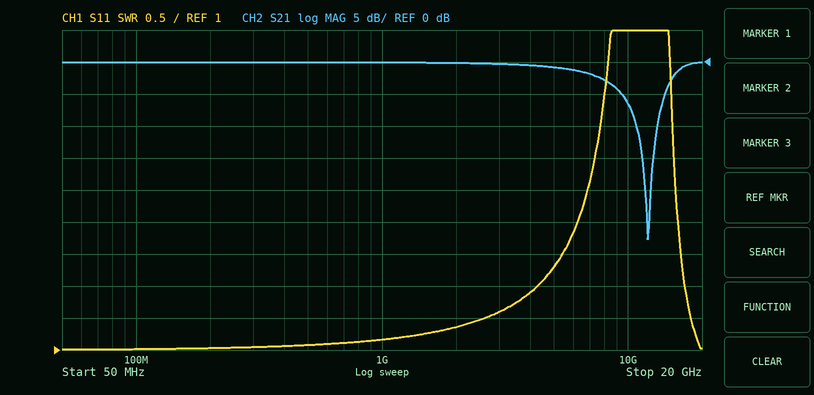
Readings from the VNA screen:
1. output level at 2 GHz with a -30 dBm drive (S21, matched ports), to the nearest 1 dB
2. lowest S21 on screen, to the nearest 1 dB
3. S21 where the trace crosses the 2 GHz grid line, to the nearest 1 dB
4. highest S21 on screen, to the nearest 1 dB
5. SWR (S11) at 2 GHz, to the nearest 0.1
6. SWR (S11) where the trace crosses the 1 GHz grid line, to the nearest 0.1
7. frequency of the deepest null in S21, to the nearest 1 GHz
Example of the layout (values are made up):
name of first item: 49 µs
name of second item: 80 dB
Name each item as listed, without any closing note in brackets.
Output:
output level at 2 GHz with a -30 dBm drive (S21, matched ports), to the nearest 1 dB: -30 dBm
lowest S21 on screen, to the nearest 1 dB: -28 dB
S21 where the trace crosses the 2 GHz grid line, to the nearest 1 dB: 0 dB
highest S21 on screen, to the nearest 1 dB: 0 dB
SWR (S11) at 2 GHz, to the nearest 0.1: 1.4
SWR (S11) where the trace crosses the 1 GHz grid line, to the nearest 0.1: 1.2
frequency of the deepest null in S21, to the nearest 1 GHz: 12 GHz
